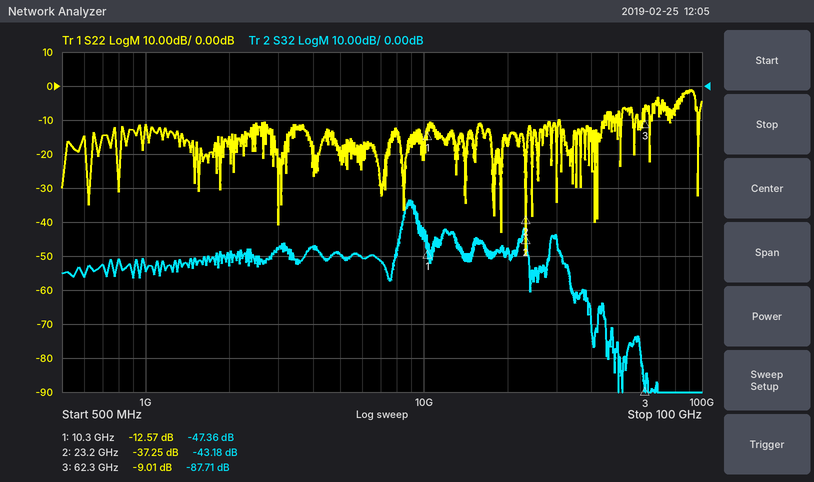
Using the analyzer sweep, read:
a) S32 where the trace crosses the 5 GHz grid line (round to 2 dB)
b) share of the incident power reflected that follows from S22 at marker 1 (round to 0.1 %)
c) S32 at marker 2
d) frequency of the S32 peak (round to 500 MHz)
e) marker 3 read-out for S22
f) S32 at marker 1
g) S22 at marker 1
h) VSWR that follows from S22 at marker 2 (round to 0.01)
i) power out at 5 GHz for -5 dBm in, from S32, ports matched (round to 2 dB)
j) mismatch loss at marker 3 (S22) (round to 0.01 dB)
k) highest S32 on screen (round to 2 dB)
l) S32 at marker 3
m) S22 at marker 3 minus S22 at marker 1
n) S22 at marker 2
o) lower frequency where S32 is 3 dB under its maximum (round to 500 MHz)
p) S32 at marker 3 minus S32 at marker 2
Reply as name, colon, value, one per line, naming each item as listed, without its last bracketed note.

S32 where the trace crosses the 5 GHz grid line: -50 dB
share of the incident power reflected that follows from S22 at marker 1: 5.5 %
S32 at marker 2: -43.18 dB
frequency of the S32 peak: 9.0 GHz
marker 3 read-out for S22: -9.01 dB
S32 at marker 1: -47.36 dB
S22 at marker 1: -12.57 dB
VSWR that follows from S22 at marker 2: 1.03
power out at 5 GHz for -5 dBm in, from S32, ports matched: -54 dBm
mismatch loss at marker 3 (S22): 0.58 dB
highest S32 on screen: -34 dB
S32 at marker 3: -87.71 dB
S22 at marker 3 minus S22 at marker 1: 3.56 dB
S22 at marker 2: -37.25 dB
lower frequency where S32 is 3 dB under its maximum: 8.5 GHz
S32 at marker 3 minus S32 at marker 2: -44.53 dB
